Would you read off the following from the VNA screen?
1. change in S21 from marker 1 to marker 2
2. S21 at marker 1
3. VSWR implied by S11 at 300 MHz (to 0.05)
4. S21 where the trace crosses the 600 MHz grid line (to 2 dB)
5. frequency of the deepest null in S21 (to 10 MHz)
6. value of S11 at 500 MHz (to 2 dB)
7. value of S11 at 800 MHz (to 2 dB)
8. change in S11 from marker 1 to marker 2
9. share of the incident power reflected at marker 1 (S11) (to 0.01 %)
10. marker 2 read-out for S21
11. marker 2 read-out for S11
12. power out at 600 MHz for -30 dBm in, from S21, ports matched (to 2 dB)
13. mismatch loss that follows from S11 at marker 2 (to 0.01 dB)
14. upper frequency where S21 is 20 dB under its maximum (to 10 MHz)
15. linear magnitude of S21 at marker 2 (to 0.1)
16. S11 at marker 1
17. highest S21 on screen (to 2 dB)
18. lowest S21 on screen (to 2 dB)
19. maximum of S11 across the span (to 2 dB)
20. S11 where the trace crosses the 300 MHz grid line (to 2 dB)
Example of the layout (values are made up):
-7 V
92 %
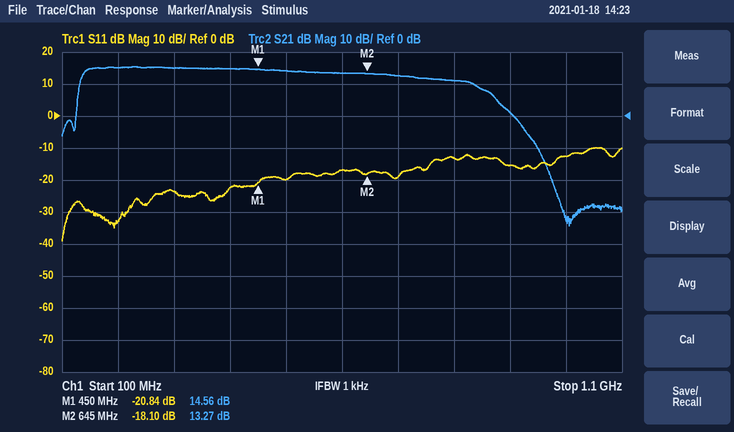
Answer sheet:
-1.29 dB
14.56 dB
1.15
14 dB
1.01 GHz
-20 dB
-14 dB
2.74 dB
0.82 %
13.27 dB
-18.10 dB
-16 dBm
0.07 dB
930 MHz
4.6
-20.84 dB
16 dB
-34 dB
-10 dB
-24 dB
